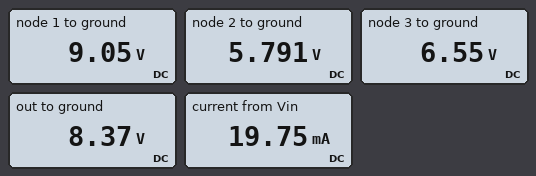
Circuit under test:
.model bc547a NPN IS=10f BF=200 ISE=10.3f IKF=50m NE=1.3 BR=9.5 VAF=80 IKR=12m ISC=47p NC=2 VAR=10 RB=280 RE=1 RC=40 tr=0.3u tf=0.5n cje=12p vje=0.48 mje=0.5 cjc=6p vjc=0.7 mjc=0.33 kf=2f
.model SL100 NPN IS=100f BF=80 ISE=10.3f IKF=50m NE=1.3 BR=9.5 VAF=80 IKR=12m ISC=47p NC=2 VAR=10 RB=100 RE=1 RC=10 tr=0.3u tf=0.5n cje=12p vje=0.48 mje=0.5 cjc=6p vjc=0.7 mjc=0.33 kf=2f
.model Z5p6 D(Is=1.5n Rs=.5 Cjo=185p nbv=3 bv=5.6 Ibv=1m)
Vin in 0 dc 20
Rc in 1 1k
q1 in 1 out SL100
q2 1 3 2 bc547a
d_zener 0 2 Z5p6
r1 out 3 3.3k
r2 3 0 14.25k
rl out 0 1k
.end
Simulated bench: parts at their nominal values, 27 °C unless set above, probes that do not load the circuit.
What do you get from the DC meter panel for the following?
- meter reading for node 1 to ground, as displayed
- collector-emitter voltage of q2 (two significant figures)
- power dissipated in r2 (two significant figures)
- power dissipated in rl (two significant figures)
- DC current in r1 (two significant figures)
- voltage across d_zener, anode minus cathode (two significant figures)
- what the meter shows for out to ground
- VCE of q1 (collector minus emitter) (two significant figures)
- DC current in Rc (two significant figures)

9.05 V
3.3 V
3.0 mW
70 mW
550 µA
-5.8 V
8.37 V
12 V
11 mA
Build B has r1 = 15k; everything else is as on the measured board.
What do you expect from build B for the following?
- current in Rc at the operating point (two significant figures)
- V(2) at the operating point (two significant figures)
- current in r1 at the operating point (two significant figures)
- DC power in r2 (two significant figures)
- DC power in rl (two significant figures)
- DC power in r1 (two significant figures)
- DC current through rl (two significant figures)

5.5 mA
5.7 V
490 µA
2.9 mW
190 mW
3.6 mW
14 mA
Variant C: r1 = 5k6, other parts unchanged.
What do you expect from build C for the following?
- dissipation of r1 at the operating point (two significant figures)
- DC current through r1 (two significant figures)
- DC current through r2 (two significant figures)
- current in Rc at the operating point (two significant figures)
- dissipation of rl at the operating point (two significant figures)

1.6 mW
540 µA
460 µA
9.8 mA
91 mW
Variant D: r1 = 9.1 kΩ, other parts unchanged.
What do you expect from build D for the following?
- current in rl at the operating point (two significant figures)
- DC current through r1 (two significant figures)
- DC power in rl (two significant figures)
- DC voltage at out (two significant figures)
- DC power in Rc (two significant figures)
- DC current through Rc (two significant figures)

11 mA
520 µA
130 mW
11 V
65 mW
8.1 mA
